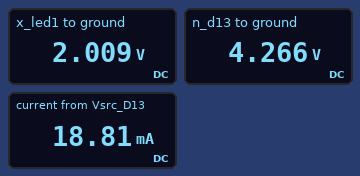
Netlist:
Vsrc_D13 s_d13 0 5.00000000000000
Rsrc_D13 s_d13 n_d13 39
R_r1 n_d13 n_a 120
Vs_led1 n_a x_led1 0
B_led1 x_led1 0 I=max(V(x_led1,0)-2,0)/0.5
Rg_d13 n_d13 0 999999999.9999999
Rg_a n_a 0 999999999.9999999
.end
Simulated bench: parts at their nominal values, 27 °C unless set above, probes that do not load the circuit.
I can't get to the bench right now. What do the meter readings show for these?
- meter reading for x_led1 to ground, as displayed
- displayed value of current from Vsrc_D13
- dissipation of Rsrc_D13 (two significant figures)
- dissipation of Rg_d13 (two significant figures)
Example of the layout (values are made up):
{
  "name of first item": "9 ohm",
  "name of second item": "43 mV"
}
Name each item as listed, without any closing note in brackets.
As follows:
{
  "meter reading for x_led1 to ground, as displayed": "2.009 V",
  "displayed value of current from Vsrc_D13": "18.81 mA",
  "dissipation of Rsrc_D13": "14 mW",
  "dissipation of Rg_d13": "18 nW"
}
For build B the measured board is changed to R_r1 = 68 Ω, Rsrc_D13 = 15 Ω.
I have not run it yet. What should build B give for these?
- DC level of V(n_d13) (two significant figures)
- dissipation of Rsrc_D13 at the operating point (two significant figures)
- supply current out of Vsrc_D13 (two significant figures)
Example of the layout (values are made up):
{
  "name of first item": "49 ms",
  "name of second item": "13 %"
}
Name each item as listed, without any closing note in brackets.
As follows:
{
  "DC level of V(n_d13)": "4.5 V",
  "dissipation of Rsrc_D13 at the operating point": "19 mW",
  "supply current out of Vsrc_D13": "36 mA"
}
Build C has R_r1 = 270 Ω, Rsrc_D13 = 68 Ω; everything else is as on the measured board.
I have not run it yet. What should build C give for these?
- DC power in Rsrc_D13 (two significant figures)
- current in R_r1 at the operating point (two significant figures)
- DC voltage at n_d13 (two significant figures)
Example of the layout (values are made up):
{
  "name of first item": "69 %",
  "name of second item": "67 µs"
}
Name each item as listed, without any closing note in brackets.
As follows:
{
  "DC power in Rsrc_D13": "5.3 mW",
  "current in R_r1 at the operating point": "8.9 mA",
  "DC voltage at n_d13": "4.4 V"
}
